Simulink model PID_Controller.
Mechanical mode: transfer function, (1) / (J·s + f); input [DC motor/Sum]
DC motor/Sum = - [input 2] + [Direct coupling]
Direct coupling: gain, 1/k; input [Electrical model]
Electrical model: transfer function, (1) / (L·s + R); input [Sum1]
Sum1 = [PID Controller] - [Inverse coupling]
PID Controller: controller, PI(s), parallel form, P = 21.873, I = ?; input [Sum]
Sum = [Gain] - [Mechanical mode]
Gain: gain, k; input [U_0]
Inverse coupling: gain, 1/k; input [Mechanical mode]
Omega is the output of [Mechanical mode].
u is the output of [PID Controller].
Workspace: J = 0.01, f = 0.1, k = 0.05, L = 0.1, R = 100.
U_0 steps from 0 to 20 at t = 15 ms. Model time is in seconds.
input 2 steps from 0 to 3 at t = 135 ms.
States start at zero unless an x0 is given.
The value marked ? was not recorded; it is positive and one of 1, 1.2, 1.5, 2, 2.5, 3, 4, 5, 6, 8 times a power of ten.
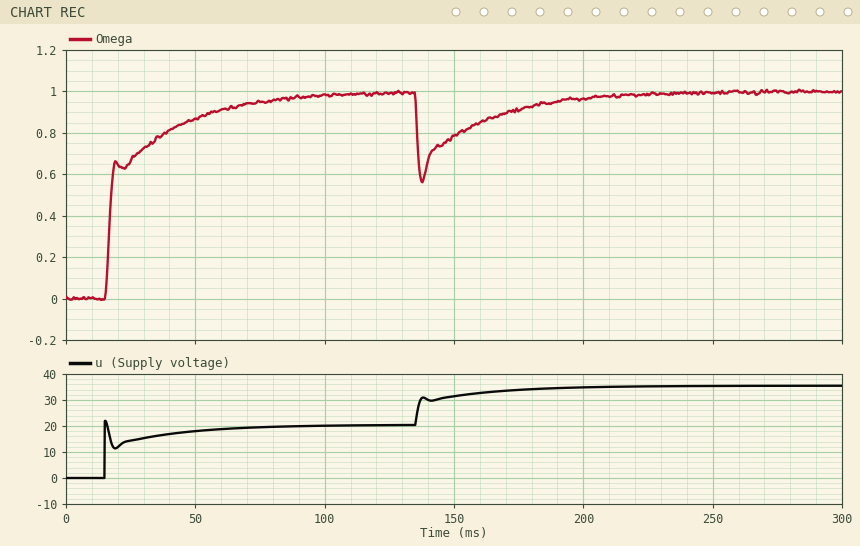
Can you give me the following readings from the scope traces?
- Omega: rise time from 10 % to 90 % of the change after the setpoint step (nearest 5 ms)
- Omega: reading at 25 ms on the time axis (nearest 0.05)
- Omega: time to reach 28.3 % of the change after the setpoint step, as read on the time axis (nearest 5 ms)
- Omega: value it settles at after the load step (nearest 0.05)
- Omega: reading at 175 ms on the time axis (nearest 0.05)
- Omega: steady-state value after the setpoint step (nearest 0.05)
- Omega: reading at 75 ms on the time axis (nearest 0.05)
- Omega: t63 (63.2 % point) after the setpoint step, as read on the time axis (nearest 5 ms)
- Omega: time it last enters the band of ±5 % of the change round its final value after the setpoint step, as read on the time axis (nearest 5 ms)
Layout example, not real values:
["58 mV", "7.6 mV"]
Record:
["40 ms", "0.65", "15 ms", "1.00", "0.90", "1.00", "0.95", "20 ms", "75 ms"]
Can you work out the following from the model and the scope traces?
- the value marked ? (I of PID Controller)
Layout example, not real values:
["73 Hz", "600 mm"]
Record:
["1500"]
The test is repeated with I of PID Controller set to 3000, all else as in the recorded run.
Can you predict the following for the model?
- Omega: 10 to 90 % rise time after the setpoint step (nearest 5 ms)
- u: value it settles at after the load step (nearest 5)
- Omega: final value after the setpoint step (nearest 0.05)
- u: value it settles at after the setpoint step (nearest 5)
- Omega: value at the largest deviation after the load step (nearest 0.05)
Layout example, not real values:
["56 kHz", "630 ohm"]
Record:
["20 ms", "35", "1.00", "20", "0.60"]
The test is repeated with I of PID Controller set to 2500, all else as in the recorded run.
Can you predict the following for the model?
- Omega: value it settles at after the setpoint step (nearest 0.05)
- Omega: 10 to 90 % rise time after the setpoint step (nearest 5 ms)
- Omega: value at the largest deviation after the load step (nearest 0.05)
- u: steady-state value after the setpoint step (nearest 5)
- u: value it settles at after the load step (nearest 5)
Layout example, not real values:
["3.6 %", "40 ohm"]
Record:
["1.00", "25 ms", "0.60", "20", "35"]
